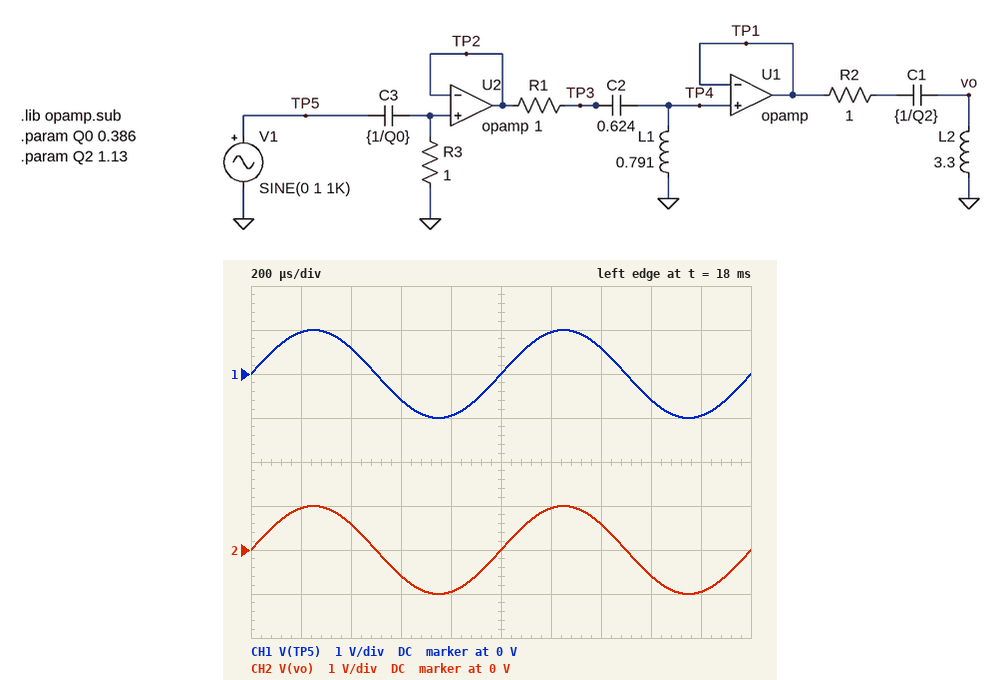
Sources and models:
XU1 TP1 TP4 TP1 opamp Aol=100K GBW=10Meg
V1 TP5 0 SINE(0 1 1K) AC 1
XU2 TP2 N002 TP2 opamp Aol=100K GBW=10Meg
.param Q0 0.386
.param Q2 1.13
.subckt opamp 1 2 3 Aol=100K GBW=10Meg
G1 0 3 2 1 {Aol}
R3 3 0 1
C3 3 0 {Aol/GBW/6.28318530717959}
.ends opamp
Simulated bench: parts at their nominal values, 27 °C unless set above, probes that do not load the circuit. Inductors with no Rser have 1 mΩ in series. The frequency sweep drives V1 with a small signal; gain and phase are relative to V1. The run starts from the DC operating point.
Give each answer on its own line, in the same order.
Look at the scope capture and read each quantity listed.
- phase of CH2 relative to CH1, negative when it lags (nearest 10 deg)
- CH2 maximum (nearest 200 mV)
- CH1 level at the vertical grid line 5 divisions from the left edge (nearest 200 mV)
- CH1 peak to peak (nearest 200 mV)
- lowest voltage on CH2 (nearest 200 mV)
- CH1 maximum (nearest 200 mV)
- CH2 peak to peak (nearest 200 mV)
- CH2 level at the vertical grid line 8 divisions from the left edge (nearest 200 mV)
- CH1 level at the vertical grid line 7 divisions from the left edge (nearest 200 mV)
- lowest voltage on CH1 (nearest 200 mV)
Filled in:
0 deg
1.0 V
0 V
2.0 V
-1.0 V
1.0 V
2.0 V
-600 mV
600 mV
-1.0 V
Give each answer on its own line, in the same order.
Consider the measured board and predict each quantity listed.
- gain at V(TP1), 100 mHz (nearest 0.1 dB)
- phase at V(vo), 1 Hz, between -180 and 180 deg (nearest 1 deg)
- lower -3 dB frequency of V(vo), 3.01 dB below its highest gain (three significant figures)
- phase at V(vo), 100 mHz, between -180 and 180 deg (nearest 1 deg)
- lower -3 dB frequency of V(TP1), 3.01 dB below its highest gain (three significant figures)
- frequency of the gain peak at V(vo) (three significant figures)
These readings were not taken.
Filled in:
-14.6 dB
18 deg
179 mHz
-100 deg
194 mHz
274 mHz
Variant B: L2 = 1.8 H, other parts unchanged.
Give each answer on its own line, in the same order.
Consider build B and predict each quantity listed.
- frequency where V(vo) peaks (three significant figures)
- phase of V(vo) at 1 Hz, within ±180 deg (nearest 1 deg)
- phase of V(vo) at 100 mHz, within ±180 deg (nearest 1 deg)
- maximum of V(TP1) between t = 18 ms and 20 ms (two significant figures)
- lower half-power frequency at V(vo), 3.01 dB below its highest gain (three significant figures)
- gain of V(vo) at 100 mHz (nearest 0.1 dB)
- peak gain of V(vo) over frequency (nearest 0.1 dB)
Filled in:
265 mHz
21 deg
-51 deg
1.0 V
175 mHz
-15.2 dB
3.1 dB
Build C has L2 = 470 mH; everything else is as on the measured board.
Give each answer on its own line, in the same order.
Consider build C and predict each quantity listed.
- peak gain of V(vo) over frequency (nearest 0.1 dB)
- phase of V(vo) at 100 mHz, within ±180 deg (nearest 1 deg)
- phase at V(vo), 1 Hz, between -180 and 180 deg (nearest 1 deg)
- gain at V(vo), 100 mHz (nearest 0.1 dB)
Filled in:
0.9 dB
-28 deg
35 deg
-30.4 dB
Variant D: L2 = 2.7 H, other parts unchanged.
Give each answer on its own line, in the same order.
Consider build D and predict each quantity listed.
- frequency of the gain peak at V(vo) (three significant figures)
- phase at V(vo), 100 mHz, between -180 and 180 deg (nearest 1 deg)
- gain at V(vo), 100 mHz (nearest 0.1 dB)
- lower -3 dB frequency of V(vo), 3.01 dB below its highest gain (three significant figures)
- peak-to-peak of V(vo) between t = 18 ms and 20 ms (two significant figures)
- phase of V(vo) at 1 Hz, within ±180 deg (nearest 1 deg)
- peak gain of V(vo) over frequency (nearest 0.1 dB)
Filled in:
271 mHz
-79 deg
-10.1 dB
177 mHz
2.0 V
19 deg
2.8 dB
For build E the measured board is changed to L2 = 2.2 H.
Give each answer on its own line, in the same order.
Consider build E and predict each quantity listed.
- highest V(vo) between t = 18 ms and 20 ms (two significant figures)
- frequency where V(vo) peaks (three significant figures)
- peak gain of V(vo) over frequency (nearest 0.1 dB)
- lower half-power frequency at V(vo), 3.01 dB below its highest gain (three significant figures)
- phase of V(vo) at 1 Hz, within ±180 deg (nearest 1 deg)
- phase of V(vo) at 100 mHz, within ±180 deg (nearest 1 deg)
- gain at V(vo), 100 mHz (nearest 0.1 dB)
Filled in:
1.0 V
267 mHz
3.0 dB
175 mHz
20 deg
-62 deg
-12.5 dB
